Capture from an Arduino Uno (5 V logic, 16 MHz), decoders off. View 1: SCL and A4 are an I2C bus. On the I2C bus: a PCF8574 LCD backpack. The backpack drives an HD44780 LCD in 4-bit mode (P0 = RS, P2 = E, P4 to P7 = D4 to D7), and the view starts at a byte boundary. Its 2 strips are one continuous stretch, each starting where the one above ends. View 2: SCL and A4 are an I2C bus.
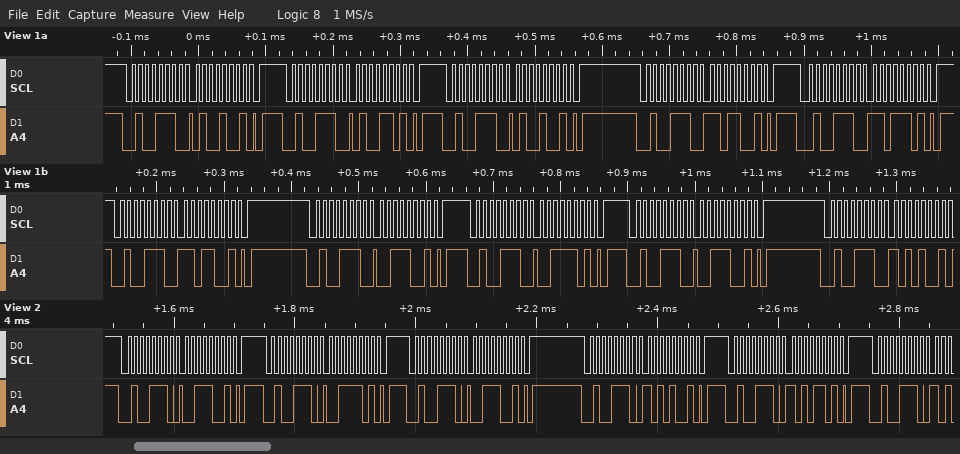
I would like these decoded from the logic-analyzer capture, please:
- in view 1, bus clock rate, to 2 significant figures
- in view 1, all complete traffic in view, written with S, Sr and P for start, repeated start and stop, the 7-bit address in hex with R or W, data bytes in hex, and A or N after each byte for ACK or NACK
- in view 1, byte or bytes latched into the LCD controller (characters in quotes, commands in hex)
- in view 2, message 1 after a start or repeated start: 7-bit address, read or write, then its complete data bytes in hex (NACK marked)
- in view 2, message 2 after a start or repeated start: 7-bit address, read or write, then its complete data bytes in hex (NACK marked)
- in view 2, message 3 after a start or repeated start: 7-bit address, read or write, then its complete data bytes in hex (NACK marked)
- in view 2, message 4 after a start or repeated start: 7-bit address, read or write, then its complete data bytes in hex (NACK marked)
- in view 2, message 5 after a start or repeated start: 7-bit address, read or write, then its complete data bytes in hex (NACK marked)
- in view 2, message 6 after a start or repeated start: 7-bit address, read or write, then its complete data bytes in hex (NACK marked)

100 kHz
S 27W A 49 A P S 27W A 4D A P S 27W A 49 A P S 27W A D9 A P S 27W A DD A P S 27W A D9 A P S 27W A 39 A P S 27W A 3D A P S 27W A 39 A P S 27W A A9 A
'M'
0x27 write: 39
0x27 write: 3D
0x27 write: 39
0x27 write: A9
0x27 write: AD
0x27 write
